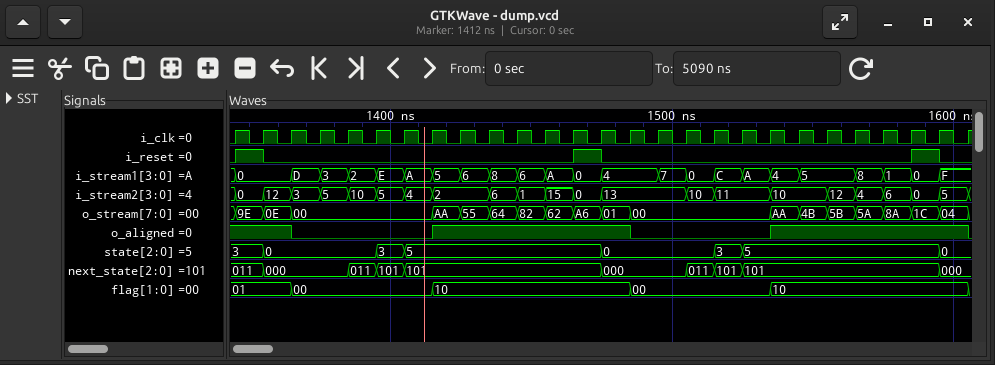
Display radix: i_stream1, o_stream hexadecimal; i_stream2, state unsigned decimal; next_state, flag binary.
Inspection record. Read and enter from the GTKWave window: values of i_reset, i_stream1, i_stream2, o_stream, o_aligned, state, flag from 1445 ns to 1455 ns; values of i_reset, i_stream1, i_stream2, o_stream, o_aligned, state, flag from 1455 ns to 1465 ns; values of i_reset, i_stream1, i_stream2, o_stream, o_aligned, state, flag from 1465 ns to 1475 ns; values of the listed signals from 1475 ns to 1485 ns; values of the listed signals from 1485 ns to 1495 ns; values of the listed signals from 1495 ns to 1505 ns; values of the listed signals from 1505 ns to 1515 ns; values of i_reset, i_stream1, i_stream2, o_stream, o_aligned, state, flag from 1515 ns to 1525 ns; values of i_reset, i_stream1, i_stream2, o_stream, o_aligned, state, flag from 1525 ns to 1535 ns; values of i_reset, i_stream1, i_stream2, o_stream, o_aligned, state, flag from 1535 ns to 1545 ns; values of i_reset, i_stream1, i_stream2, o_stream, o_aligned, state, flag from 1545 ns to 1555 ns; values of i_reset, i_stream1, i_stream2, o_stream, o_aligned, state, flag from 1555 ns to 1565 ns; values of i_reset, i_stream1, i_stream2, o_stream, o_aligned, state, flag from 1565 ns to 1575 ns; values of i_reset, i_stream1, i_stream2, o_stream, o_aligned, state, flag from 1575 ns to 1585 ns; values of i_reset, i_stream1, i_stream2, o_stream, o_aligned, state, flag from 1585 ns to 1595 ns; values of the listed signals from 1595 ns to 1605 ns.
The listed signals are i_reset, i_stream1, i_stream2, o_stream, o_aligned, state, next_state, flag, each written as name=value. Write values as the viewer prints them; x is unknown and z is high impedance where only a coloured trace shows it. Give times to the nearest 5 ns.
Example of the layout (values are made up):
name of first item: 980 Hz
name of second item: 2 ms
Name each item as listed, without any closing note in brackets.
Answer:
values of i_reset, i_stream1, i_stream2, o_stream, o_aligned, state, flag from 1445 ns to 1455 ns: i_reset=0, i_stream1=6, i_stream2=1, o_stream=82, o_aligned=1, state=5, flag=10
values of i_reset, i_stream1, i_stream2, o_stream, o_aligned, state, flag from 1455 ns to 1465 ns: i_reset=0, i_stream1=A, i_stream2=15, o_stream=62, o_aligned=1, state=5, flag=10
values of i_reset, i_stream1, i_stream2, o_stream, o_aligned, state, flag from 1465 ns to 1475 ns: i_reset=1, i_stream1=0, i_stream2=0, o_stream=A6, o_aligned=1, state=5, flag=10
values of the listed signals from 1475 ns to 1485 ns: i_reset=0, i_stream1=4, i_stream2=13, o_stream=01, o_aligned=1, state=0, next_state=000, flag=10
values of the listed signals from 1485 ns to 1495 ns: i_reset=0, i_stream1=4, i_stream2=13, o_stream=00, o_aligned=0, state=0, next_state=000, flag=00
values of the listed signals from 1495 ns to 1505 ns: i_reset=0, i_stream1=7, i_stream2=13, o_stream=00, o_aligned=0, state=0, next_state=000, flag=00
values of the listed signals from 1505 ns to 1515 ns: i_reset=0, i_stream1=0, i_stream2=10, o_stream=00, o_aligned=0, state=0, next_state=011, flag=00
values of i_reset, i_stream1, i_stream2, o_stream, o_aligned, state, flag from 1515 ns to 1525 ns: i_reset=0, i_stream1=C, i_stream2=11, o_stream=00, o_aligned=0, state=3, flag=00
values of i_reset, i_stream1, i_stream2, o_stream, o_aligned, state, flag from 1525 ns to 1535 ns: i_reset=0, i_stream1=A, i_stream2=11, o_stream=00, o_aligned=0, state=5, flag=00
values of i_reset, i_stream1, i_stream2, o_stream, o_aligned, state, flag from 1535 ns to 1545 ns: i_reset=0, i_stream1=4, i_stream2=10, o_stream=AA, o_aligned=1, state=5, flag=10
values of i_reset, i_stream1, i_stream2, o_stream, o_aligned, state, flag from 1545 ns to 1555 ns: i_reset=0, i_stream1=5, i_stream2=10, o_stream=4B, o_aligned=1, state=5, flag=10
values of i_reset, i_stream1, i_stream2, o_stream, o_aligned, state, flag from 1555 ns to 1565 ns: i_reset=0, i_stream1=5, i_stream2=12, o_stream=5B, o_aligned=1, state=5, flag=10
values of i_reset, i_stream1, i_stream2, o_stream, o_aligned, state, flag from 1565 ns to 1575 ns: i_reset=0, i_stream1=8, i_stream2=4, o_stream=5A, o_aligned=1, state=5, flag=10
values of i_reset, i_stream1, i_stream2, o_stream, o_aligned, state, flag from 1575 ns to 1585 ns: i_reset=0, i_stream1=1, i_stream2=6, o_stream=8A, o_aligned=1, state=5, flag=10
values of i_reset, i_stream1, i_stream2, o_stream, o_aligned, state, flag from 1585 ns to 1595 ns: i_reset=1, i_stream1=0, i_stream2=0, o_stream=1C, o_aligned=1, state=5, flag=10
values of the listed signals from 1595 ns to 1605 ns: i_reset=0, i_stream1=F, i_stream2=5, o_stream=04, o_aligned=1, state=0, next_state=000, flag=10
